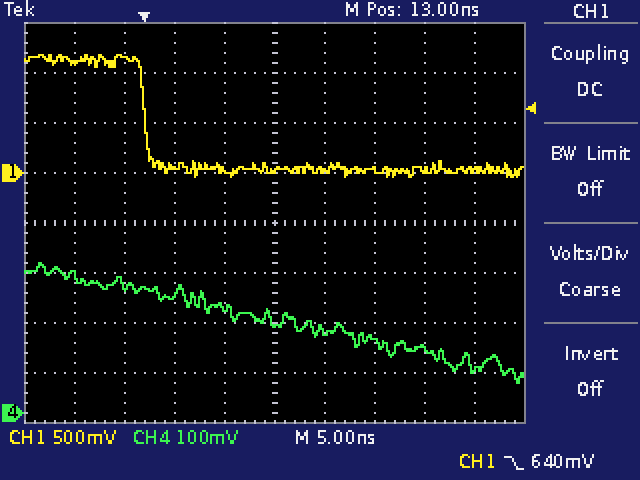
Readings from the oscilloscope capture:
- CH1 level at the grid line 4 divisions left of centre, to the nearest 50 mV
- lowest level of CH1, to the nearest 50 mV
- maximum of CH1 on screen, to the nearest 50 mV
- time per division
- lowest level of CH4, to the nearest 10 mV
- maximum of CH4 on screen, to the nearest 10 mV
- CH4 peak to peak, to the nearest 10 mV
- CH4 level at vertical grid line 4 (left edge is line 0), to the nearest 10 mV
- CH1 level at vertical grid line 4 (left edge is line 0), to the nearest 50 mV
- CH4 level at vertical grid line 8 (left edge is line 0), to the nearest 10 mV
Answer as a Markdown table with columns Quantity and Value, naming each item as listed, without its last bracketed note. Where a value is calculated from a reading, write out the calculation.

| Quantity | Value |
|---|---|
| CH1 level at the grid line 4 divisions left of centre, to the nearest 50 mV | 1.10 V |
| lowest level of CH1, to the nearest 50 mV | -50 mV |
| maximum of CH1 on screen, to the nearest 50 mV | 1.20 V |
| time per division | 5 ns |
| lowest level of CH4, to the nearest 10 mV | 60 mV |
| maximum of CH4 on screen, to the nearest 10 mV | 300 mV |
| CH4 peak to peak, to the nearest 10 mV | 300 mV − (60 mV) = 240 mV |
| CH4 level at vertical grid line 4 (left edge is line 0), to the nearest 10 mV | 210 mV |
| CH1 level at vertical grid line 4 (left edge is line 0), to the nearest 50 mV | 50 mV |
| CH4 level at vertical grid line 8 (left edge is line 0), to the nearest 10 mV | 130 mV |
